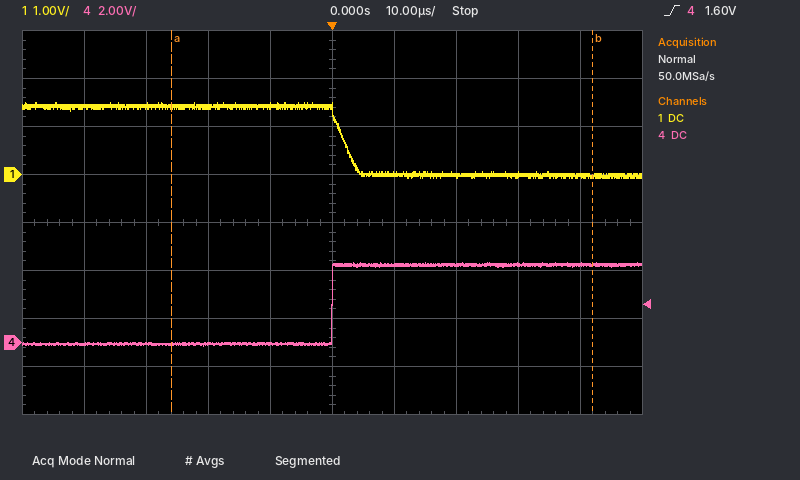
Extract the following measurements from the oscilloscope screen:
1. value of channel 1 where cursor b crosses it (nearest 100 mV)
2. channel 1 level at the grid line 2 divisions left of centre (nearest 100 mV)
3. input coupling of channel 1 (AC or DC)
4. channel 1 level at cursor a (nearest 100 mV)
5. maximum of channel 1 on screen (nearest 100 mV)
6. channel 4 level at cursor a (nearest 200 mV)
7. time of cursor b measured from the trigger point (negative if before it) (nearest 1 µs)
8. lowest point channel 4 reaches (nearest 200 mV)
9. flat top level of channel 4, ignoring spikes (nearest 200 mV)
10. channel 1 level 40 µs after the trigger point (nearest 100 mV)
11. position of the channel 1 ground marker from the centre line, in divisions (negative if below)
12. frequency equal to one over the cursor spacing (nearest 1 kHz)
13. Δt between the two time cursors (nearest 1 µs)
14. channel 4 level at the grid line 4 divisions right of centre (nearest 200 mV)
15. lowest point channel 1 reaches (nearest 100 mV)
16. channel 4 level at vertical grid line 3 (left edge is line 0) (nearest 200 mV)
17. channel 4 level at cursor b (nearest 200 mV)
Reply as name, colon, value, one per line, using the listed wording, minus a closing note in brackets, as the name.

value of channel 1 where cursor b crosses it: 0.0 V
channel 1 level at the grid line 2 divisions left of centre: 1.4 V
input coupling of channel 1: DC
channel 1 level at cursor a: 1.4 V
maximum of channel 1 on screen: 1.5 V
channel 4 level at cursor a: 0.0 V
time of cursor b measured from the trigger point (negative if before it): +42 µs
lowest point channel 4 reaches: -200 mV
flat top level of channel 4, ignoring spikes: 3.2 V
channel 1 level 40 µs after the trigger point: 0.0 V
position of the channel 1 ground marker from the centre line, in divisions: +1.0 div
frequency equal to one over the cursor spacing: 15 kHz
Δt between the two time cursors: 68 µs
channel 4 level at the grid line 4 divisions right of centre: 3.2 V
lowest point channel 1 reaches: -100 mV
channel 4 level at vertical grid line 3 (left edge is line 0): 0.0 V
channel 4 level at cursor b: 3.2 V
